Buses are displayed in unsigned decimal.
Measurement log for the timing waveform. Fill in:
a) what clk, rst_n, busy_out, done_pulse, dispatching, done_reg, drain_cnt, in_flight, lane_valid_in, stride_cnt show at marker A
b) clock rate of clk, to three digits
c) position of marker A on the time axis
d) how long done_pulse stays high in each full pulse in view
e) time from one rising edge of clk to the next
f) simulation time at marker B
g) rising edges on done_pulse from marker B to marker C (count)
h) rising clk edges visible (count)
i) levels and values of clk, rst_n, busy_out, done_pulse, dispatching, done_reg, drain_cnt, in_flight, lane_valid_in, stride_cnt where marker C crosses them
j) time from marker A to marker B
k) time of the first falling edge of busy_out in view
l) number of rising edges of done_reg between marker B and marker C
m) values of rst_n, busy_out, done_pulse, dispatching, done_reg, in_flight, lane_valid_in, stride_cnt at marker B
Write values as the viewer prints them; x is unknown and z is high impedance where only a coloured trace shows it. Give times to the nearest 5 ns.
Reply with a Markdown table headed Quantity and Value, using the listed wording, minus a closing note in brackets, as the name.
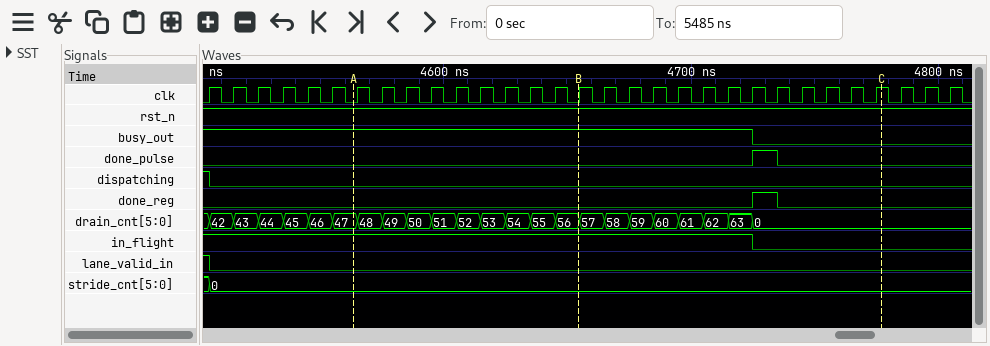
| Quantity | Value |
|---|---|
| what clk, rst_n, busy_out, done_pulse, dispatching, done_reg, drain_cnt, in_flight, lane_valid_in, stride_cnt show at marker A | clk=0, rst_n=1, busy_out=1, done_pulse=0, dispatching=0, done_reg=0, drain_cnt=47, in_flight=1, lane_valid_in=0, stride_cnt=0 |
| clock rate of clk, to three digits | 100 MHz |
| position of marker A on the time axis | 4565 ns |
| how long done_pulse stays high in each full pulse in view | 10 ns |
| time from one rising edge of clk to the next | 10 ns |
| simulation time at marker B | 4655 ns |
| rising edges on done_pulse from marker B to marker C | 1 |
| rising clk edges visible | 31 |
| levels and values of clk, rst_n, busy_out, done_pulse, dispatching, done_reg, drain_cnt, in_flight, lane_valid_in, stride_cnt where marker C crosses them | clk=1, rst_n=1, busy_out=0, done_pulse=0, dispatching=0, done_reg=0, drain_cnt=0, in_flight=0, lane_valid_in=0, stride_cnt=0 |
| time from marker A to marker B | 90 ns |
| time of the first falling edge of busy_out in view | 4725 ns |
| number of rising edges of done_reg between marker B and marker C | 1 |
| values of rst_n, busy_out, done_pulse, dispatching, done_reg, in_flight, lane_valid_in, stride_cnt at marker B | rst_n=1, busy_out=1, done_pulse=0, dispatching=0, done_reg=0, in_flight=1, lane_valid_in=0, stride_cnt=0 |
